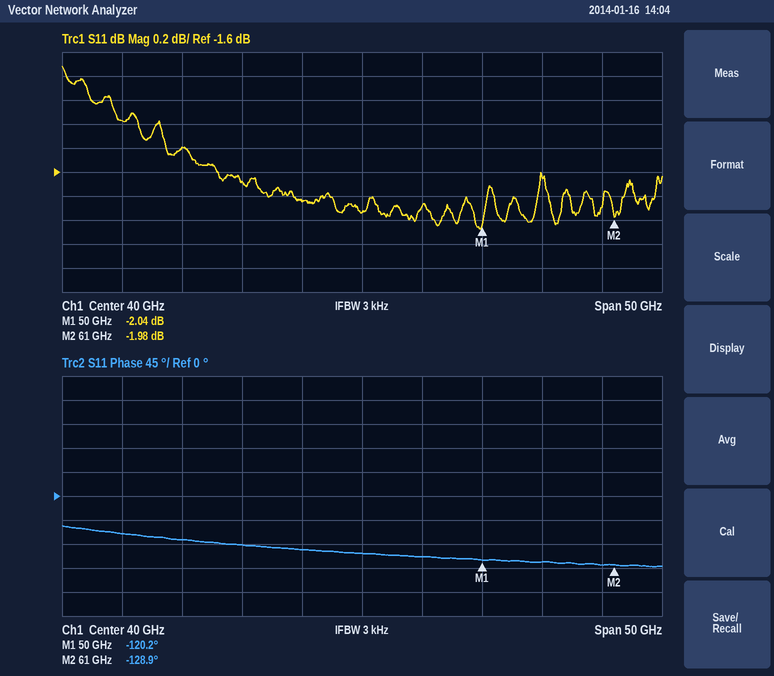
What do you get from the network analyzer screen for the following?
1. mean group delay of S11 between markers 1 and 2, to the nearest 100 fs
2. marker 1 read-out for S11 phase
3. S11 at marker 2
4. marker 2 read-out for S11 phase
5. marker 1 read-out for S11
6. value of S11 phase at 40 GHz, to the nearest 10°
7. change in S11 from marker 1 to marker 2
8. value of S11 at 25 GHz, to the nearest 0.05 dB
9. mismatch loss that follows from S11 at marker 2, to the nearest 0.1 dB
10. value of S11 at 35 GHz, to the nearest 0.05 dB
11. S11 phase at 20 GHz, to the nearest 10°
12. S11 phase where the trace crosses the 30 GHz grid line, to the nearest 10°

2.2 ps
-120.2°
-1.98 dB
-128.9°
-2.04 dB
-110°
0.06 dB
-1.40 dB
4.4 dB
-1.85 dB
-70°
-90°
